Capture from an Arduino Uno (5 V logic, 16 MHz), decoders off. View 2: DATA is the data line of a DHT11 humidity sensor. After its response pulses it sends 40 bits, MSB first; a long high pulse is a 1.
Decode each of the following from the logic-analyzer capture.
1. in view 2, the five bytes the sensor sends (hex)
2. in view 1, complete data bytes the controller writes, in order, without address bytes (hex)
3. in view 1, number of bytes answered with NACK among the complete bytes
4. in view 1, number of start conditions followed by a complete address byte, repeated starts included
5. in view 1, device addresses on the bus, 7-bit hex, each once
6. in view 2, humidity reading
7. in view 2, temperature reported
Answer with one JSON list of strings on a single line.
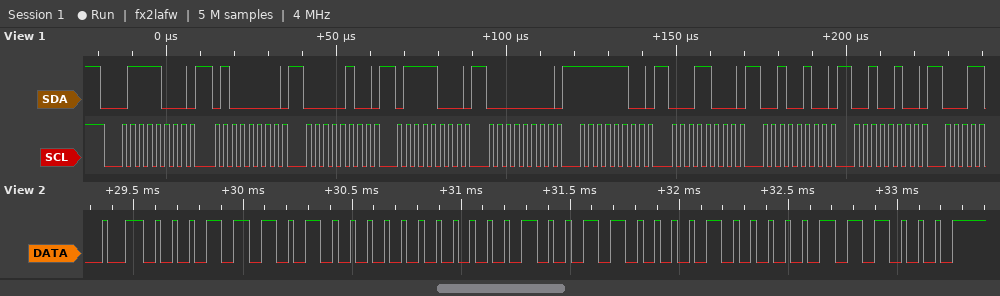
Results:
["1D 00 13 08 38", "40 04 78 00 FC 18 24 24", "0", "1", "0x3C", "29 %", "19.8 °C"]
